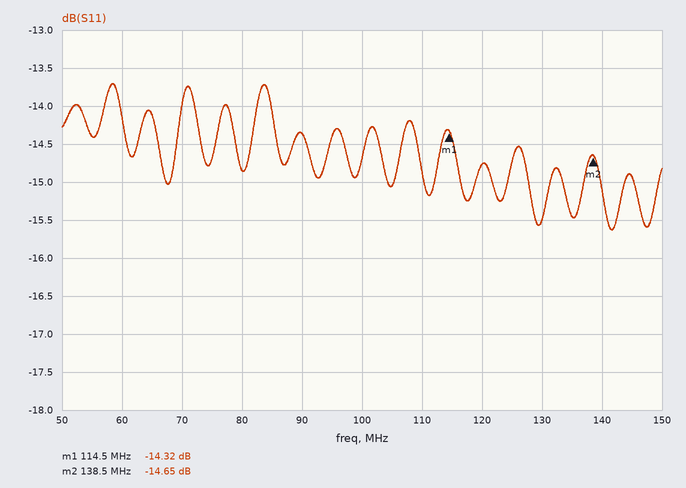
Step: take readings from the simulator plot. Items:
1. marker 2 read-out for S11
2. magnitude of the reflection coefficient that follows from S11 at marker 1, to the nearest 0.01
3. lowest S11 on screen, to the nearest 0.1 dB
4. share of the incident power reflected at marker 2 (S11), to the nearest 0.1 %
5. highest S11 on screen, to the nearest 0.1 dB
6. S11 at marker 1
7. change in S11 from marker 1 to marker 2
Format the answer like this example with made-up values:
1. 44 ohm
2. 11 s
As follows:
1. -14.65 dB
2. 0.19
3. -15.6 dB
4. 3.4 %
5. -13.7 dB
6. -14.32 dB
7. -0.33 dB
